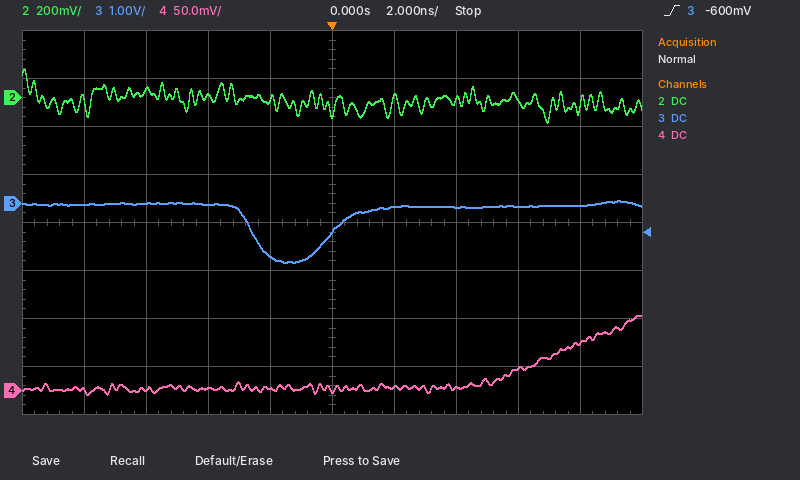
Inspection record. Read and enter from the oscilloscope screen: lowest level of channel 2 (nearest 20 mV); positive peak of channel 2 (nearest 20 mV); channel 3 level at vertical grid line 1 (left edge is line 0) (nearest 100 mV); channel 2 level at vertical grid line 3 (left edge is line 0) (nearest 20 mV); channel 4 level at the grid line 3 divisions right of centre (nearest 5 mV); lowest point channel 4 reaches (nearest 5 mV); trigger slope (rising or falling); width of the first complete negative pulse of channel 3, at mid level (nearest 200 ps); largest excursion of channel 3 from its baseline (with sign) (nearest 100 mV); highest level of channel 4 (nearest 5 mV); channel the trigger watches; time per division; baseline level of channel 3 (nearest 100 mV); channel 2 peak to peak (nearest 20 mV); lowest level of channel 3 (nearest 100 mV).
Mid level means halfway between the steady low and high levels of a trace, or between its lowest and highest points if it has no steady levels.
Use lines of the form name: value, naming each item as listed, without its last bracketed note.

lowest level of channel 2: -100 mV
positive peak of channel 2: 120 mV
channel 3 level at vertical grid line 1 (left edge is line 0): 0.0 V
channel 2 level at vertical grid line 3 (left edge is line 0): 0 mV
channel 4 level at the grid line 3 divisions right of centre: 25 mV
lowest point channel 4 reaches: -5 mV
trigger slope: rising
width of the first complete negative pulse of channel 3, at mid level: 2.6 ns
largest excursion of channel 3 from its baseline (with sign): -1.2 V
highest level of channel 4: 80 mV
channel the trigger watches: channel 3
time per division: 2 ns
baseline level of channel 3: 0.0 V
channel 2 peak to peak: 220 mV
lowest level of channel 3: -1.2 V
